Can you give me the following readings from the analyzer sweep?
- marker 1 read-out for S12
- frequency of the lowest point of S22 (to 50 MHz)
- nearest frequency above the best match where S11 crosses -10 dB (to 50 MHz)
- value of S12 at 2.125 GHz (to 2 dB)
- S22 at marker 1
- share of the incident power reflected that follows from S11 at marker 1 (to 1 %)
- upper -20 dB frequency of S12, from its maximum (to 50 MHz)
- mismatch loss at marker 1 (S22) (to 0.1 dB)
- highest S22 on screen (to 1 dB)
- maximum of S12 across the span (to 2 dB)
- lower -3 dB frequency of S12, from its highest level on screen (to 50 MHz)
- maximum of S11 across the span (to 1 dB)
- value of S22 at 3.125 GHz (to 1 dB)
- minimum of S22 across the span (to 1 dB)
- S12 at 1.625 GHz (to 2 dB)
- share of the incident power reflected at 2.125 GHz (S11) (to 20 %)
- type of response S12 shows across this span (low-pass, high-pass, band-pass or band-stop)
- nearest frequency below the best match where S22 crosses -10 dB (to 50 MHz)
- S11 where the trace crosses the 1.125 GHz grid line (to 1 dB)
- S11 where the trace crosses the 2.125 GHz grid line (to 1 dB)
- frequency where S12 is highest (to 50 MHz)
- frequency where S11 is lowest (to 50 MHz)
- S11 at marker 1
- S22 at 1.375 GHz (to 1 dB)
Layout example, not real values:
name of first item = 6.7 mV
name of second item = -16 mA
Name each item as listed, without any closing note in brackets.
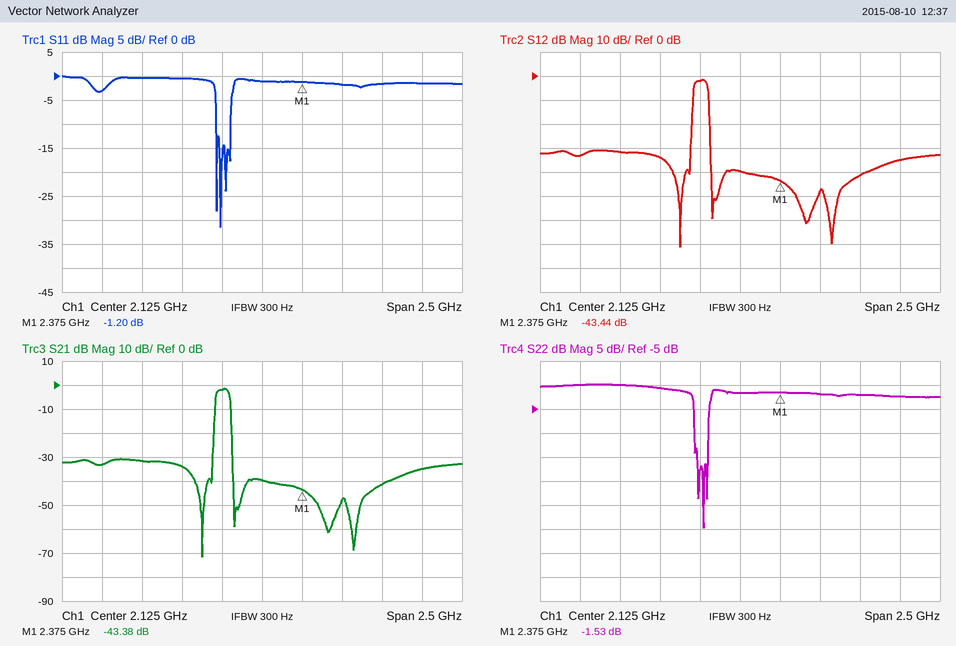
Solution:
marker 1 read-out for S12 = -43.44 dB
frequency of the lowest point of S22 = 1.90 GHz
nearest frequency above the best match where S11 crosses -10 dB = 1.95 GHz
value of S12 at 2.125 GHz = -40 dB
S22 at marker 1 = -1.53 dB
share of the incident power reflected that follows from S11 at marker 1 = 76 %
upper -20 dB frequency of S12, from its maximum = 1.95 GHz
mismatch loss at marker 1 (S22) = 5.3 dB
highest S22 on screen = 0 dB
maximum of S12 across the span = -2 dB
lower -3 dB frequency of S12, from its highest level on screen = 1.85 GHz
maximum of S11 across the span = 0 dB
value of S22 at 3.125 GHz = -2 dB
minimum of S22 across the span = -30 dB
S12 at 1.625 GHz = -34 dB
share of the incident power reflected at 2.125 GHz (S11) = 80 %
type of response S12 shows across this span = band-pass
nearest frequency below the best match where S22 crosses -10 dB = 1.85 GHz
S11 where the trace crosses the 1.125 GHz grid line = -3 dB
S11 where the trace crosses the 2.125 GHz grid line = -1 dB
frequency where S12 is highest = 1.90 GHz
frequency where S11 is lowest = 1.85 GHz
S11 at marker 1 = -1.20 dB
S22 at 1.375 GHz = 0 dB
